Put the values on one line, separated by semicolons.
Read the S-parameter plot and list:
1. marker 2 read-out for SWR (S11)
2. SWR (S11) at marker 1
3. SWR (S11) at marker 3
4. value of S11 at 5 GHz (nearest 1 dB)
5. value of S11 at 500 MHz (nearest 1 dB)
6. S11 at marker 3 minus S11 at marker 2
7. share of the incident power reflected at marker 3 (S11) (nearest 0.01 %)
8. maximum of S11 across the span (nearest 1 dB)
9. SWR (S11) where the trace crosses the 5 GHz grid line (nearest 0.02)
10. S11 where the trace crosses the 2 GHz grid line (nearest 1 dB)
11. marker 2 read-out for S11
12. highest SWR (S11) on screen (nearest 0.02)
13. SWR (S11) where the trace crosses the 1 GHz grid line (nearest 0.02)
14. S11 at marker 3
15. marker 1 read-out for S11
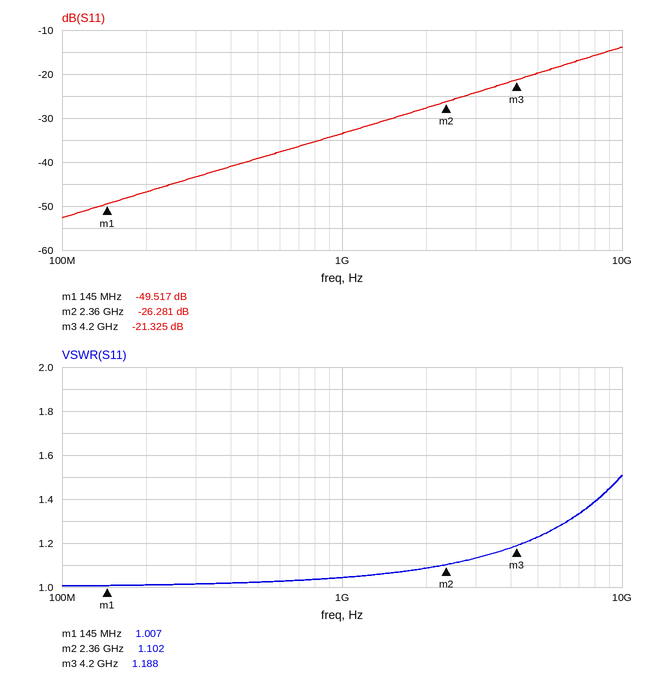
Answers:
1.102; 1.007; 1.188; -20 dB; -39 dB; 4.956 dB; 0.74 %; -14 dB; 1.22; -28 dB; -26.281 dB; 1.50; 1.04; -21.325 dB; -49.517 dB
